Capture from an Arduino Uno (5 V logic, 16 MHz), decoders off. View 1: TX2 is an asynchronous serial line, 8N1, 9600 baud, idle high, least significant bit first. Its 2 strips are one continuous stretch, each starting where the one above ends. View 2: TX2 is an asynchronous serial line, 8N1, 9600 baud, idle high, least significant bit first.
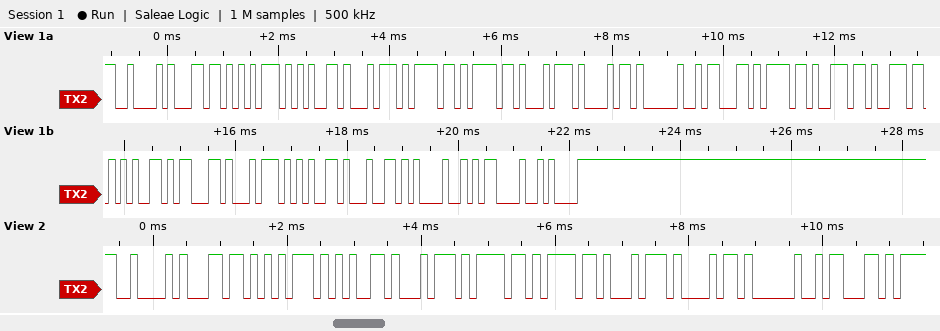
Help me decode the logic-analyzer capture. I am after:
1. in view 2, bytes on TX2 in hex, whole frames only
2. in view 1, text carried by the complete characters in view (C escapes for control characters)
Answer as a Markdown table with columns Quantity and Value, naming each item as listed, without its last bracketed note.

| Quantity | Value |
|---|---|
| in view 2, bytes on TX2 in hex, whole frames only | 42 6C 75 65 74 6F 6F 74 68 20 63 |
| in view 1, text carried by the complete characters in view | "Bluetooth connected!\r\n" |
